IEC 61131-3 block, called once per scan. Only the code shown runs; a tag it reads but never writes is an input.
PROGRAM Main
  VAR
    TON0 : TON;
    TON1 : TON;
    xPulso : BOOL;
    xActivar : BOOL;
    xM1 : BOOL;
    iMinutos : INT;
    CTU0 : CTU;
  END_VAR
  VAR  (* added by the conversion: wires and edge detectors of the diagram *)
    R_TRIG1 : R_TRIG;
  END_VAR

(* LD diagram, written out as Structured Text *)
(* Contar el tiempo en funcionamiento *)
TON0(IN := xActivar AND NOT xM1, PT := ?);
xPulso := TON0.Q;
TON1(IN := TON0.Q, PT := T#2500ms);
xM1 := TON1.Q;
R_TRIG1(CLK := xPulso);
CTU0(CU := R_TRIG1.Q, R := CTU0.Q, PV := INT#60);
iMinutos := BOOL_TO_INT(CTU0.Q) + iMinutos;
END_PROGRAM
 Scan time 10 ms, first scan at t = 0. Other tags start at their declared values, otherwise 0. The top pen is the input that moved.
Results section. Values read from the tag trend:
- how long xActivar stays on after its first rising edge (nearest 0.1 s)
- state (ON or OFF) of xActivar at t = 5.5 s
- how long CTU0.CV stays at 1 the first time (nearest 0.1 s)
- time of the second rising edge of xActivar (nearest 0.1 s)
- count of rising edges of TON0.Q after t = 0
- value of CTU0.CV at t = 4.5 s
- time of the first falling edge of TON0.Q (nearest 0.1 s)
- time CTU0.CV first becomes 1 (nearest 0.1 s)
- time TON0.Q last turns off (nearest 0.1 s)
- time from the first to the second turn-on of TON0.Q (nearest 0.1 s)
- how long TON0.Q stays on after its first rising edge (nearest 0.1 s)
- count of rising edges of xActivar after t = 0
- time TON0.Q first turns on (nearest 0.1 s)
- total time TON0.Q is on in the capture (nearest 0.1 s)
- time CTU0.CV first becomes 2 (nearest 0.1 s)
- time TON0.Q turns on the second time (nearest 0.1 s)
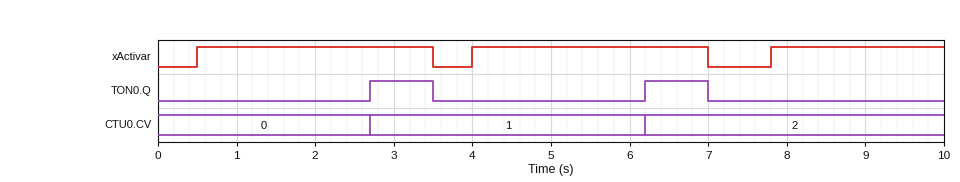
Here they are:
3.0 s
ON
3.5 s
4.0 s
2
1
3.5 s
2.7 s
7.0 s
3.5 s
0.8 s
3
2.7 s
1.6 s
6.2 s
6.2 s
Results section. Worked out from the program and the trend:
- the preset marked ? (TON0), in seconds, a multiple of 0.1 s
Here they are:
2.2 s
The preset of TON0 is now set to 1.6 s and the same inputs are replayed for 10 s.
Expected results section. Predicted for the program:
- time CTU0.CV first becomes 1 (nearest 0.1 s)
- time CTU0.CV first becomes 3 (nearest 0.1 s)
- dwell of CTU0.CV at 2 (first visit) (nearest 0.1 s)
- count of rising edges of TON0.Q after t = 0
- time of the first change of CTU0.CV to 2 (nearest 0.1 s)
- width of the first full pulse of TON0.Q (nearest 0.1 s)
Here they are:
2.1 s
9.4 s
3.8 s
3
5.6 s
1.4 s
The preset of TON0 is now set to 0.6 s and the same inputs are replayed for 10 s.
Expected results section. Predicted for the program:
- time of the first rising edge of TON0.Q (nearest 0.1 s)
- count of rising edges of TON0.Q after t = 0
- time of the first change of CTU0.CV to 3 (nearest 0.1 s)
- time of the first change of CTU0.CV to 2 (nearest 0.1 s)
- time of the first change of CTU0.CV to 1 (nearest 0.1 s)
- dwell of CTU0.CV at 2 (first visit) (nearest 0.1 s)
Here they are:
1.1 s
3
8.4 s
4.6 s
1.1 s
3.8 s
